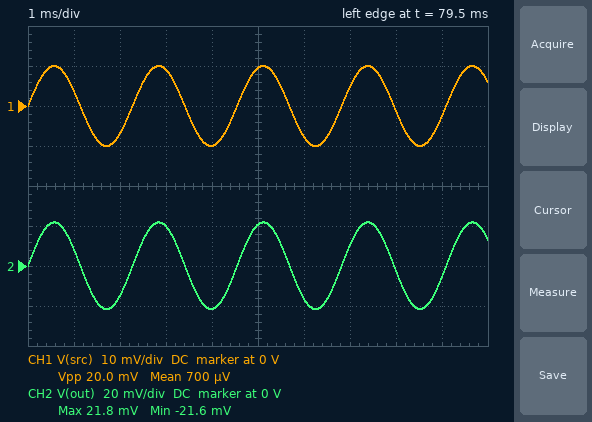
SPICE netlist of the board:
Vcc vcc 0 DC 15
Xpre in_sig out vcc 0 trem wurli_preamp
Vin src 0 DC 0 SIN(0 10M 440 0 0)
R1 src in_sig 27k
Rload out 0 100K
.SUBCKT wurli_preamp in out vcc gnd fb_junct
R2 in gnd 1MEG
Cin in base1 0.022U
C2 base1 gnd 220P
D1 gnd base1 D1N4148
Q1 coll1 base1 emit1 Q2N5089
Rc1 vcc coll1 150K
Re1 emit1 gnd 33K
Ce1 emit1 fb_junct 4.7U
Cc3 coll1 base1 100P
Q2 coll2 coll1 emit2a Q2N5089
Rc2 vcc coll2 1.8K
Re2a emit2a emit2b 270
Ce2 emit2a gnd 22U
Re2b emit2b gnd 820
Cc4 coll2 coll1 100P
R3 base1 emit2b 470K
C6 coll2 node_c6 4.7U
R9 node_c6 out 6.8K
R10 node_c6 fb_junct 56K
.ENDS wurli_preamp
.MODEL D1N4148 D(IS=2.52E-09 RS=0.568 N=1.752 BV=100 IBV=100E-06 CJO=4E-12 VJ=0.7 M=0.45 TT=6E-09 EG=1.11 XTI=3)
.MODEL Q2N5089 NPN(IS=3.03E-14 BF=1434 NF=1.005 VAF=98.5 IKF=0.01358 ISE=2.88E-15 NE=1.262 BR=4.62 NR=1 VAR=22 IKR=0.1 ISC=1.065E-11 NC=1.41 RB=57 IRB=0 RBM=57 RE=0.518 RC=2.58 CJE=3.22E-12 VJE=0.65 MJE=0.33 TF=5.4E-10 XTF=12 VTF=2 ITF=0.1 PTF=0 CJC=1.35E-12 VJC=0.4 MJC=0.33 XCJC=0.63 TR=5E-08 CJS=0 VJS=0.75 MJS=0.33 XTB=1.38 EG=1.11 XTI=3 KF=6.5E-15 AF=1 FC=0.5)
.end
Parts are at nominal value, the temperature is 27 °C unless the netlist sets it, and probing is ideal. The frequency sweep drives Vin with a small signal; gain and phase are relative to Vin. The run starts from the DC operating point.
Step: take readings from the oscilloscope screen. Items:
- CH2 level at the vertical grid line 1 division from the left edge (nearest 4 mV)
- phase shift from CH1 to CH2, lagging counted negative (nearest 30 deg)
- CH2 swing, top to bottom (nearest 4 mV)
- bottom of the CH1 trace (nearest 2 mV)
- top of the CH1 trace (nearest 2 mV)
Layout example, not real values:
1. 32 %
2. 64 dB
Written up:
1. 8 mV
2. 0 deg
3. 44 mV
4. -10 mV
5. 10 mV
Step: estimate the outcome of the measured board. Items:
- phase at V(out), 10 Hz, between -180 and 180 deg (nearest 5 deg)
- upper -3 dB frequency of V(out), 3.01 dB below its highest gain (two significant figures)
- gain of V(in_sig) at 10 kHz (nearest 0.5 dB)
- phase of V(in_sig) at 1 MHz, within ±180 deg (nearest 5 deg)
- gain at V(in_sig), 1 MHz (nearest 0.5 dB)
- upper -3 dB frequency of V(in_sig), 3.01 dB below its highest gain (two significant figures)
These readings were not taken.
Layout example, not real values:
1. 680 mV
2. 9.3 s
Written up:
1. 85 deg
2. 16 kHz
3. -1.5 dB
4. -90 deg
5. -34.5 dB
6. 18 kHz
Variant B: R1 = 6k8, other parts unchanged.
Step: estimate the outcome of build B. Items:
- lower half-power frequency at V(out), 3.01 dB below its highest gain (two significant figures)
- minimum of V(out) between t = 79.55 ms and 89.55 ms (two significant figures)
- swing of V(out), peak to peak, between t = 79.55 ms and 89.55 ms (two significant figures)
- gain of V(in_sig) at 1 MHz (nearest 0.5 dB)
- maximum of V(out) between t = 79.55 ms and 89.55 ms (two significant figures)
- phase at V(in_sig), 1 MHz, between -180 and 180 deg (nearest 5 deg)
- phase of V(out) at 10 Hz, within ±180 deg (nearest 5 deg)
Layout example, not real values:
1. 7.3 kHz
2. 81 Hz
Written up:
1. 15 Hz
2. -23 mV
3. 46 mV
4. -22.5 dB
5. 23 mV
6. -85 deg
7. 90 deg
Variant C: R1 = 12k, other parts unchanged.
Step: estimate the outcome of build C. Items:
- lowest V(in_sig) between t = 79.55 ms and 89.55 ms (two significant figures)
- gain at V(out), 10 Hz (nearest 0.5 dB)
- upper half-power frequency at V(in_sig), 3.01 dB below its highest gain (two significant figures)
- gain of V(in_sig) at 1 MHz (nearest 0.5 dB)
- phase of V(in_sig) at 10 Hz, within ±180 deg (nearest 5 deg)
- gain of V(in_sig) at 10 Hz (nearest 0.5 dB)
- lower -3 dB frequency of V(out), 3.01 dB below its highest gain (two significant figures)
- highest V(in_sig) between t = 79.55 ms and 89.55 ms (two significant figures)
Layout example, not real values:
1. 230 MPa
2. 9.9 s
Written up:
1. -9.6 mV
2. 0.5 dB
3. 41 kHz
4. -27.5 dB
5. 0 deg
6. 0 dB
7. 15 Hz
8. 9.6 mV
